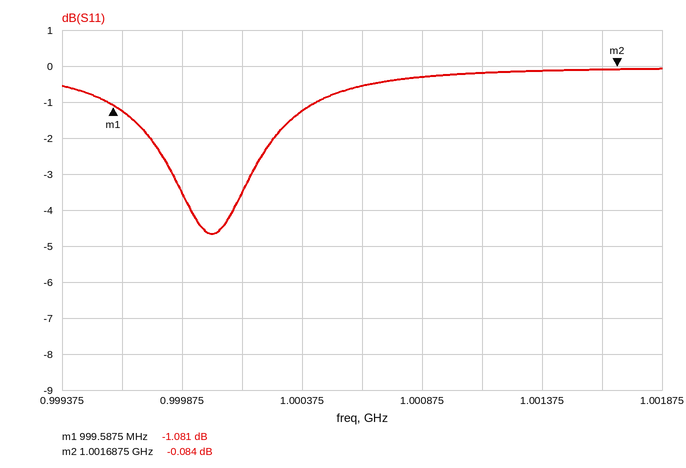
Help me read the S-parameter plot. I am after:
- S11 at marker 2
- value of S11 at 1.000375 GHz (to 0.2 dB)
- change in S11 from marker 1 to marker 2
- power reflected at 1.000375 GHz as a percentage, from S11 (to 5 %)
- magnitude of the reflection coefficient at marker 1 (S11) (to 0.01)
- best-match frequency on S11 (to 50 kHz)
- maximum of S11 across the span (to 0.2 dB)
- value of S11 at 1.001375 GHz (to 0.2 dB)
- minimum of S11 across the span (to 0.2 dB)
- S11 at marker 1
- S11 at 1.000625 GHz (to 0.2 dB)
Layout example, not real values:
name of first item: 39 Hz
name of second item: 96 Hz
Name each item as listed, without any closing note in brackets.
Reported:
S11 at marker 2: -0.084 dB
value of S11 at 1.000375 GHz: -1.2 dB
change in S11 from marker 1 to marker 2: 0.997 dB
power reflected at 1.000375 GHz as a percentage, from S11: 75 %
magnitude of the reflection coefficient at marker 1 (S11): 0.88
best-match frequency on S11: 1.00000 GHz
maximum of S11 across the span: 0.0 dB
value of S11 at 1.001375 GHz: -0.2 dB
minimum of S11 across the span: -4.6 dB
S11 at marker 1: -1.081 dB
S11 at 1.000625 GHz: -0.6 dB
